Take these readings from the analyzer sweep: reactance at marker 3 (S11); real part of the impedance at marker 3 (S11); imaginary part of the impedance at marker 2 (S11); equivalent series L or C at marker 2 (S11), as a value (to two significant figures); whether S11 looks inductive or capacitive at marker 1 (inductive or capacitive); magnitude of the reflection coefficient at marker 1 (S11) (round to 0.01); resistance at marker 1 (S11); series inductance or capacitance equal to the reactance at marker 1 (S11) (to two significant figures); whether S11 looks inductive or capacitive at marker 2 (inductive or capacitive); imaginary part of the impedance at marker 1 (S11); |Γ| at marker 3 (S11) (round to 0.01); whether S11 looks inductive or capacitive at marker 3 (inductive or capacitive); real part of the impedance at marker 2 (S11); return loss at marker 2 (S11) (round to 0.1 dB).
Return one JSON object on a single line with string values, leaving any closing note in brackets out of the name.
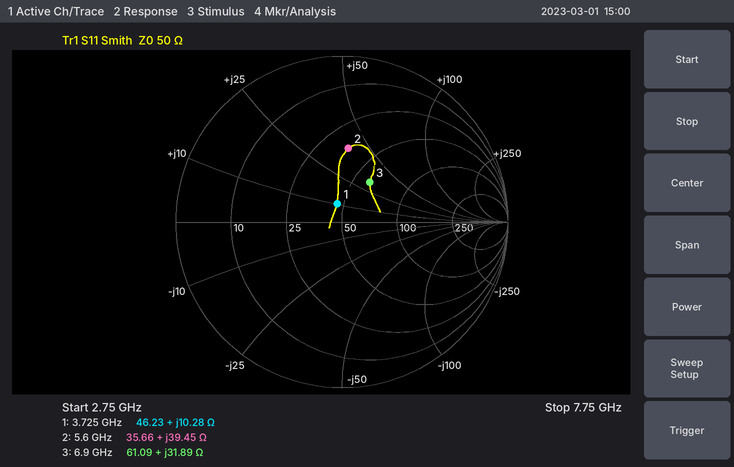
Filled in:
{"reactance at marker 3": "+31.89 Ω", "real part of the impedance at marker 3": "61.09 Ω", "imaginary part of the impedance at marker 2": "+39.45 Ω", "equivalent series L or C at marker 2 (S11), as a value": "1.1 nH", "whether S11 looks inductive or capacitive at marker 1": "inductive", "magnitude of the reflection coefficient at marker 1 (S11)": "0.11", "resistance at marker 1": "46.23 Ω", "series inductance or capacitance equal to the reactance at marker 1 (S11)": "440 pH", "whether S11 looks inductive or capacitive at marker 2": "inductive", "imaginary part of the impedance at marker 1": "+10.28 Ω", "|Γ| at marker 3 (S11)": "0.29", "whether S11 looks inductive or capacitive at marker 3": "inductive", "real part of the impedance at marker 2": "35.66 Ω", "return loss at marker 2 (S11)": "7.0 dB"}
